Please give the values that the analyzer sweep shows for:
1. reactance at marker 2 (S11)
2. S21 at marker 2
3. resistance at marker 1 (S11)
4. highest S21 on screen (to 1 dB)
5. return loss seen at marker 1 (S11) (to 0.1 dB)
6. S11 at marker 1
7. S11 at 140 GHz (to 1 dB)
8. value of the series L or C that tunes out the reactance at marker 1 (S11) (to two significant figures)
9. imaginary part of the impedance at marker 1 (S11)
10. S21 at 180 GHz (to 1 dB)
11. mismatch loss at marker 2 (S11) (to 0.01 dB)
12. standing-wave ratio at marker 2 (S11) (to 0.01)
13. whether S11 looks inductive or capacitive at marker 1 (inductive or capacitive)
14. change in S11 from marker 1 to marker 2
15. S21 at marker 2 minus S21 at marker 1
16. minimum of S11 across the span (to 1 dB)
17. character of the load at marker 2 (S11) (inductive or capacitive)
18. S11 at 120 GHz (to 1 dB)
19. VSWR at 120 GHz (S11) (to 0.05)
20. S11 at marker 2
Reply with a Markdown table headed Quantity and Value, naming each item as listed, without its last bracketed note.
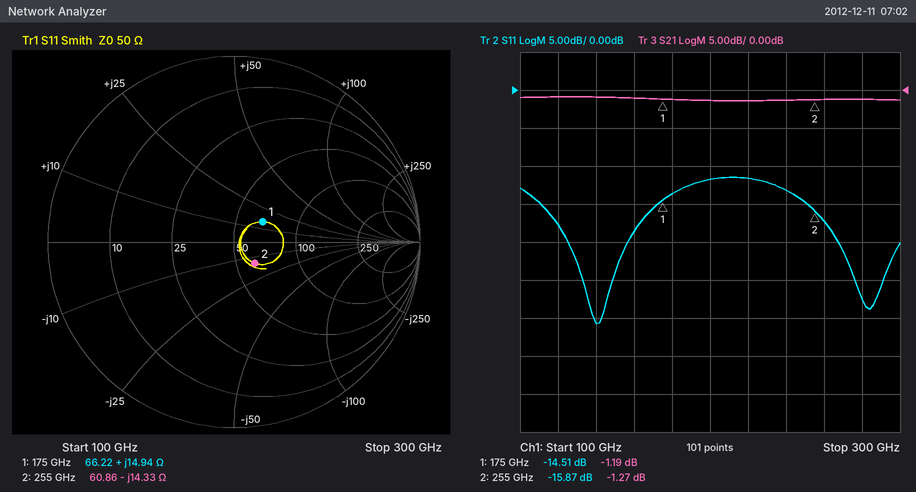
| Quantity | Value |
|---|---|
| reactance at marker 2 | -14.33 Ω |
| S21 at marker 2 | -1.27 dB |
| resistance at marker 1 | 66.22 Ω |
| highest S21 on screen | -1 dB |
| return loss seen at marker 1 (S11) | 14.5 dB |
| S11 at marker 1 | -14.51 dB |
| S11 at 140 GHz | -31 dB |
| value of the series L or C that tunes out the reactance at marker 1 (S11) | 61 fF |
| imaginary part of the impedance at marker 1 | +14.94 Ω |
| S21 at 180 GHz | -1 dB |
| mismatch loss at marker 2 (S11) | 0.11 dB |
| standing-wave ratio at marker 2 (S11) | 1.38 |
| whether S11 looks inductive or capacitive at marker 1 | inductive |
| change in S11 from marker 1 to marker 2 | -1.36 dB |
| S21 at marker 2 minus S21 at marker 1 | -0.08 dB |
| minimum of S11 across the span | -31 dB |
| character of the load at marker 2 (S11) | capacitive |
| S11 at 120 GHz | -18 dB |
| VSWR at 120 GHz (S11) | 1.30 |
| S11 at marker 2 | -15.87 dB |
